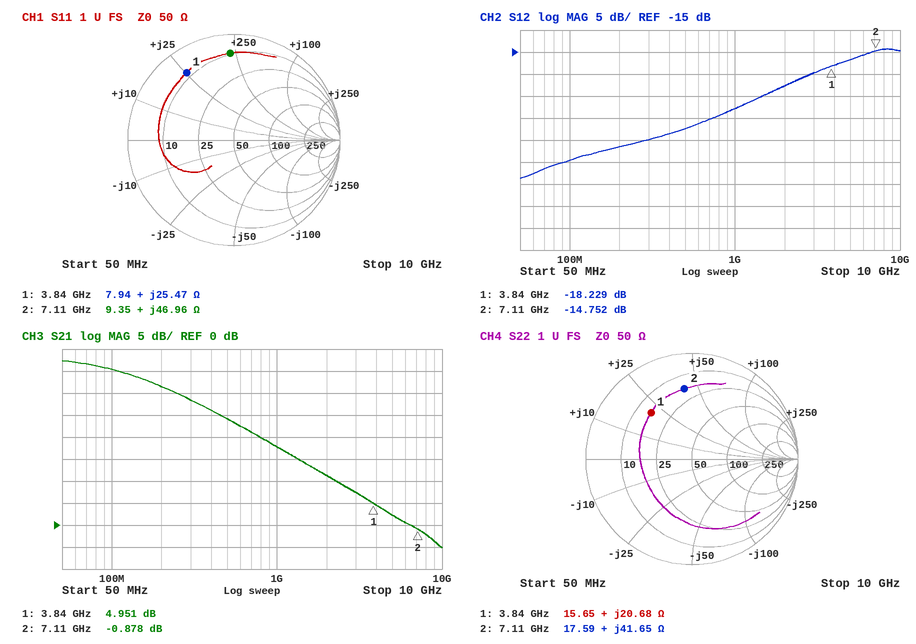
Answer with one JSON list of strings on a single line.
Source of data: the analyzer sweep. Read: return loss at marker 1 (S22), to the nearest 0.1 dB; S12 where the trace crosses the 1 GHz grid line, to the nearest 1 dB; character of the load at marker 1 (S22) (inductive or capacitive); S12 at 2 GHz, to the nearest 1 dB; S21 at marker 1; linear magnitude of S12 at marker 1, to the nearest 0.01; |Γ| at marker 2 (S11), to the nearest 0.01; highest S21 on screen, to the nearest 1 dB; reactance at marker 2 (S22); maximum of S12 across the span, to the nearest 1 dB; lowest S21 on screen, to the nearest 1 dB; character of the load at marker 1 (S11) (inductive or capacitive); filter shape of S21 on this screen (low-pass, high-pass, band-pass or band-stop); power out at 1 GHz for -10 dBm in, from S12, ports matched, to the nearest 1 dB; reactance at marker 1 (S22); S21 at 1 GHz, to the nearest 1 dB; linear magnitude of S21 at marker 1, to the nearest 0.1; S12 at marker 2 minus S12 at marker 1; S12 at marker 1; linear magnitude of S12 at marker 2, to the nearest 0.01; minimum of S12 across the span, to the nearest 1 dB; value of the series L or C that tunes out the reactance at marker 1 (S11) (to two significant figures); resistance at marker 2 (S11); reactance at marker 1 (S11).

["4.7 dB", "-28 dB", "inductive", "-23 dB", "4.951 dB", "0.12", "0.82", "37 dB", "+41.65 Ω", "-14 dB", "-5 dB", "inductive", "low-pass", "-38 dBm", "+20.68 Ω", "18 dB", "1.8", "3.477 dB", "-18.229 dB", "0.18", "-44 dB", "1.6 pF", "9.35 Ω", "+25.47 Ω"]
